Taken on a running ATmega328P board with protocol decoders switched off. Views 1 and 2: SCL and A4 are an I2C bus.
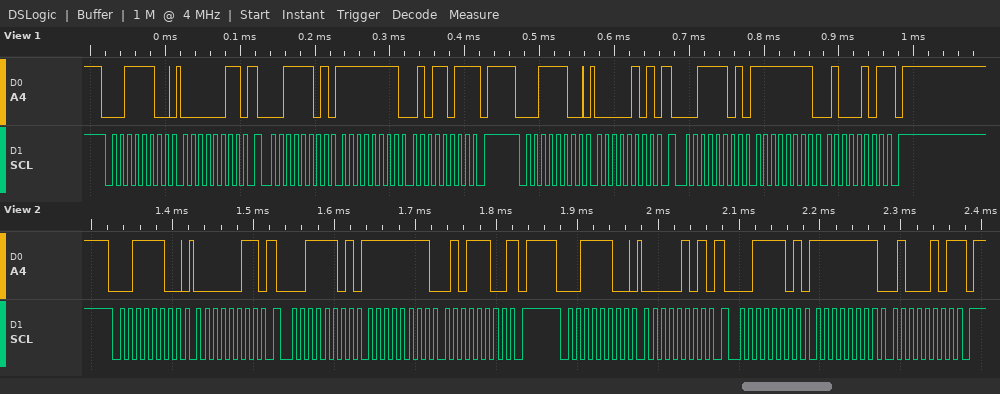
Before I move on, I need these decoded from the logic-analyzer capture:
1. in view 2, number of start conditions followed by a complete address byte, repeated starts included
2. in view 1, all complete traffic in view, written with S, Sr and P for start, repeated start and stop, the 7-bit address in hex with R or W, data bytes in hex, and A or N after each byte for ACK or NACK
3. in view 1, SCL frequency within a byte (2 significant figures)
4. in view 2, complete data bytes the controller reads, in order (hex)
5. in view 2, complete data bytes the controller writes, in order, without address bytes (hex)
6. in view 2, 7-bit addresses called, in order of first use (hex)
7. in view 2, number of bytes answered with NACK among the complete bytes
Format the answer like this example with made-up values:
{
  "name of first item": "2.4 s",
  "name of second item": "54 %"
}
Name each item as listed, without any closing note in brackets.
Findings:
{
  "in view 2, number of start conditions followed by a complete address byte, repeated starts included": "4",
  "in view 1, all complete traffic in view, written with S, Sr and P for start, repeated start and stop, the 7-bit address in hex with R or W, data bytes in hex, and A or N after each byte for ACK or NACK": "S 1EW A 03 A Sr 1ER A FF A 5B N P S 1EW A 05 A Sr 1ER A FF A 45 N P",
  "in view 1, SCL frequency within a byte": "100 kHz",
  "in view 2, complete data bytes the controller reads, in order": "FF 5C FF 45",
  "in view 2, complete data bytes the controller writes, in order, without address bytes": "03 05",
  "in view 2, 7-bit addresses called, in order of first use": "0x1E",
  "in view 2, number of bytes answered with NACK among the complete bytes": "2"
}
